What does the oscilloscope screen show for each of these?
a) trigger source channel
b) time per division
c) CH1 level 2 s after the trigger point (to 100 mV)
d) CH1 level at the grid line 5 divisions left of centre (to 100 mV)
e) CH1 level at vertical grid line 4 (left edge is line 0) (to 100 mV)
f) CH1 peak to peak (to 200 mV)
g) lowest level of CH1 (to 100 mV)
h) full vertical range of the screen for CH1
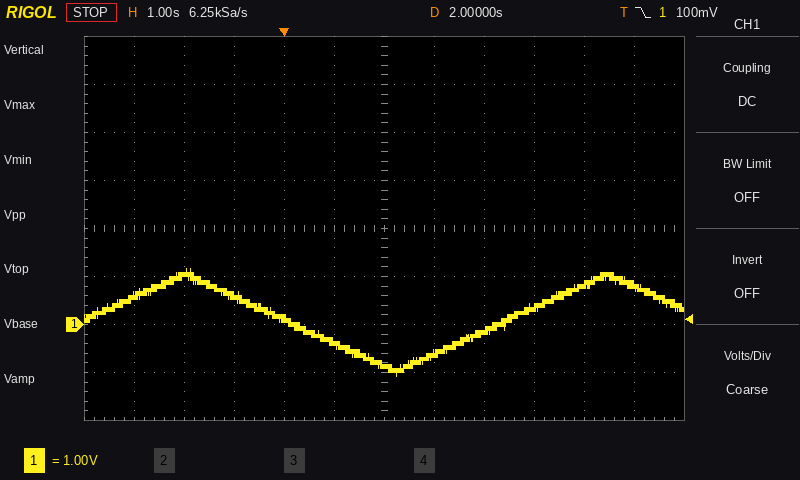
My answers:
CH1
1 s
-800 mV
600 mV
100 mV
2.2 V
-1.1 V
8 V
